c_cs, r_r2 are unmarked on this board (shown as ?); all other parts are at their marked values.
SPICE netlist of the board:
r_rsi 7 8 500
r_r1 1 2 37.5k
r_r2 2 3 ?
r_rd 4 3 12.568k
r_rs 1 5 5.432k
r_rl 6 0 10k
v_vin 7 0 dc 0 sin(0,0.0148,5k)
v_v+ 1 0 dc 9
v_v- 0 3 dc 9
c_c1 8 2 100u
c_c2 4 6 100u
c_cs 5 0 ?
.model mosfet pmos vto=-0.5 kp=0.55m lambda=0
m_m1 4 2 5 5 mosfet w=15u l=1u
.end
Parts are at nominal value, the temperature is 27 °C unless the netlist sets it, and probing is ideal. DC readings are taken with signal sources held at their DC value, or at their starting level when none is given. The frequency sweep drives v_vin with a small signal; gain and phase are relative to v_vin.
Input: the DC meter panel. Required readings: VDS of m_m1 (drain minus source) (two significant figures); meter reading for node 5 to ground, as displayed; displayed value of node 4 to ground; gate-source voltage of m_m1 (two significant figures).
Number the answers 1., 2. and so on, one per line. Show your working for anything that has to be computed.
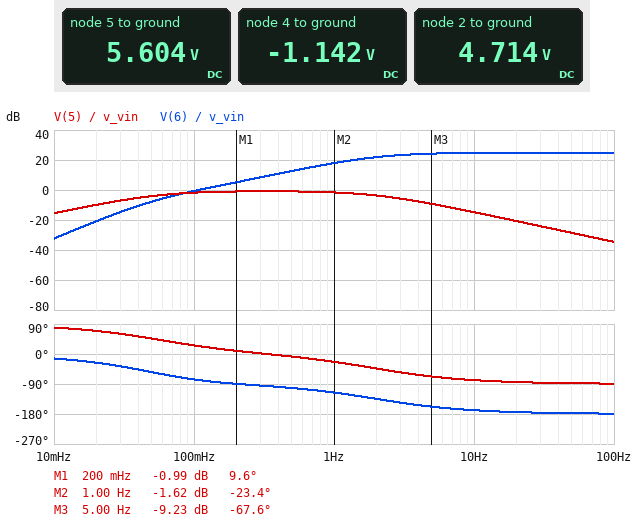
1. -1.142 V - 5.604 V = -6.7 V
2. 5.604 V
3. -1.142 V
4. 4.714 V - 5.604 V = -890 mV
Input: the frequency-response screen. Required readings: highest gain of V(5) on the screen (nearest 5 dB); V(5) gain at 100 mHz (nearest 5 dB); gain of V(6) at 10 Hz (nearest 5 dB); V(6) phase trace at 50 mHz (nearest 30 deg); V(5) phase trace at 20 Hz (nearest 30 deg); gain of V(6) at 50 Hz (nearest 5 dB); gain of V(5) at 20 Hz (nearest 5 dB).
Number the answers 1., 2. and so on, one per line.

1. 0 dB
2. 0 dB
3. 25 dB
4. -60 deg
5. -90 deg
6. 25 dB
7. -20 dB
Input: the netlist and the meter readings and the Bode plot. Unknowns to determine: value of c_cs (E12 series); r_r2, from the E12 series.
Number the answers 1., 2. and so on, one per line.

1. 270 µF
2. 120 kΩ
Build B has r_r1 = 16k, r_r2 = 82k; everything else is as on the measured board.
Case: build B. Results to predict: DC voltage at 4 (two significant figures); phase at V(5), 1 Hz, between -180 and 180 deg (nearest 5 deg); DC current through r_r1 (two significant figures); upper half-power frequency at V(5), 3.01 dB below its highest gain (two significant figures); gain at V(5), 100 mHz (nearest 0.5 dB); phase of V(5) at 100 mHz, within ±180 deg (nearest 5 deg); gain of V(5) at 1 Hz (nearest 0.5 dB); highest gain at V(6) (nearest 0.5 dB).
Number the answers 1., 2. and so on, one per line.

1. -4.1 V
2. -25 deg
3. 180 µA
4. 1.8 Hz
5. -4.5 dB
6. 45 deg
7. -2.5 dB
8. 22.5 dB
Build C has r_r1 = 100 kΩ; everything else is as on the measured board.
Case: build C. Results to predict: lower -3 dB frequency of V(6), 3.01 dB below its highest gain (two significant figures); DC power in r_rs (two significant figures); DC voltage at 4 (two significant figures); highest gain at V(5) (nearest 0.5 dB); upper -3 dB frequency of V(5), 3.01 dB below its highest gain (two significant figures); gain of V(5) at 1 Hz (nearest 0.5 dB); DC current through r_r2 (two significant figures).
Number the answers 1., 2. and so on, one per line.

1. 280 mHz
2. 5.4 mW
3. 3.5 V
4. -42.5 dB
5. 380 mHz
6. -52.5 dB
7. 82 µA
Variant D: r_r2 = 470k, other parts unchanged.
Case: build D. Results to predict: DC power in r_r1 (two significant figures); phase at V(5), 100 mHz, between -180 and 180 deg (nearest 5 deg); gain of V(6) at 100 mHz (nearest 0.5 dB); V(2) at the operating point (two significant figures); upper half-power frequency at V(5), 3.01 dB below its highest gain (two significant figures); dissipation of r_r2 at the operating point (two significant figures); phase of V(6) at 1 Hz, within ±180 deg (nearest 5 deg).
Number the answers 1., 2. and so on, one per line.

1. 47 µW
2. 20 deg
3. -1.0 dB
4. 7.7 V
5. 1.0 Hz
6. 590 µW
7. -135 deg
